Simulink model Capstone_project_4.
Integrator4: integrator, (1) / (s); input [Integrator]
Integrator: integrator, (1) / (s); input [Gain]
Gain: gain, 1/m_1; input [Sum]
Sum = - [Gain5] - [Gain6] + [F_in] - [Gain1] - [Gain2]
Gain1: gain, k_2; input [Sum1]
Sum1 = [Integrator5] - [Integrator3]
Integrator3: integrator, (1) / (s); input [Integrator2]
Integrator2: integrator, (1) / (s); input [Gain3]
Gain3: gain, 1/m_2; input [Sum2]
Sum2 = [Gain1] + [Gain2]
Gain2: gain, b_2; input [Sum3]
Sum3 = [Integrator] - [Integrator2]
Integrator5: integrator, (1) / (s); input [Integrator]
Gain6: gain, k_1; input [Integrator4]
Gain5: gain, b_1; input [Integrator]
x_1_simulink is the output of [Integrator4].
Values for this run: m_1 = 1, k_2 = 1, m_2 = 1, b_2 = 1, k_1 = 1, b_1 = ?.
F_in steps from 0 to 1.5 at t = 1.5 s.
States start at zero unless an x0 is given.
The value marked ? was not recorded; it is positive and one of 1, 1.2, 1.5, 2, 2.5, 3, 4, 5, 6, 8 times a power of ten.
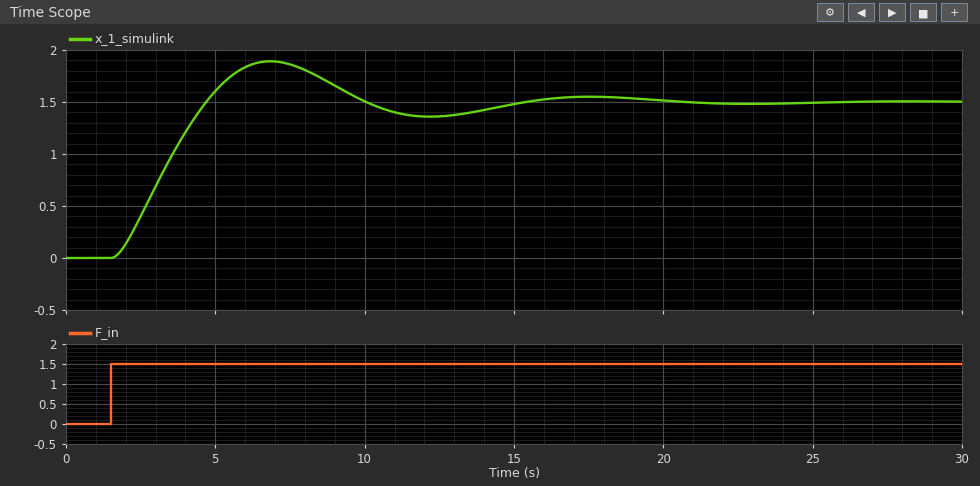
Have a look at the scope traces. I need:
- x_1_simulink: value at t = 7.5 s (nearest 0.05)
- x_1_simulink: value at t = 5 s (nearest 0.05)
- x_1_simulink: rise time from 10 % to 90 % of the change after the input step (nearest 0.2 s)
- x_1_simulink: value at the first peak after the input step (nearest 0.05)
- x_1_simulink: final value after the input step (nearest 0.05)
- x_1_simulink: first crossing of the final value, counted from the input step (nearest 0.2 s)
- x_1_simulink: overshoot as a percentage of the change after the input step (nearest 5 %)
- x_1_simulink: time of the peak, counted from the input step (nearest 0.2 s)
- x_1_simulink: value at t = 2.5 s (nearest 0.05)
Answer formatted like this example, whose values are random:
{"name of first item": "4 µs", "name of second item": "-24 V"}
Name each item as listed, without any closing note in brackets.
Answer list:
{"x_1_simulink: value at t = 7.5 s": "1.85", "x_1_simulink: value at t = 5 s": "1.60", "x_1_simulink: rise time from 10 % to 90 % of the change after the input step": "2.2 s", "x_1_simulink: value at the first peak after the input step": "1.90", "x_1_simulink: final value after the input step": "1.50", "x_1_simulink: first crossing of the final value, counted from the input step": "3.2 s", "x_1_simulink: overshoot as a percentage of the change after the input step": "25 %", "x_1_simulink: time of the peak, counted from the input step": "5.4 s", "x_1_simulink: value at t = 2.5 s": "0.40"}
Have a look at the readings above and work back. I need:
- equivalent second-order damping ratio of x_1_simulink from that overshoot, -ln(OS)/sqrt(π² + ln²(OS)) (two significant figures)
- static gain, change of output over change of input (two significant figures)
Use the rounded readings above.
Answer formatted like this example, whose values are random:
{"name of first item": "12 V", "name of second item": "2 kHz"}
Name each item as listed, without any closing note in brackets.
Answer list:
{"equivalent second-order damping ratio of x_1_simulink from that overshoot, -ln(OS)/sqrt(π² + ln²(OS))": "0.40", "static gain, change of output over change of input": "1.0"}
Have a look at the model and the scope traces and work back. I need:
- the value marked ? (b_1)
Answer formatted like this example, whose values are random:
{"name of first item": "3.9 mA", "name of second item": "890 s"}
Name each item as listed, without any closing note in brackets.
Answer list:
{"the value marked ?": "1"}
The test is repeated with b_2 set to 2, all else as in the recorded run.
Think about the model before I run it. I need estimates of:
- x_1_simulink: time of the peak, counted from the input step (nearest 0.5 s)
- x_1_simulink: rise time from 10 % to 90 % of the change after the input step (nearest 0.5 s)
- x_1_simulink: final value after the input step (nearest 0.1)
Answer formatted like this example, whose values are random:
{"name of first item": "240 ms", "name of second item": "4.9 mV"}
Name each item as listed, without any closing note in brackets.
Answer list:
{"x_1_simulink: time of the peak, counted from the input step": "5.0 s", "x_1_simulink: rise time from 10 % to 90 % of the change after the input step": "2.0 s", "x_1_simulink: final value after the input step": "1.5"}
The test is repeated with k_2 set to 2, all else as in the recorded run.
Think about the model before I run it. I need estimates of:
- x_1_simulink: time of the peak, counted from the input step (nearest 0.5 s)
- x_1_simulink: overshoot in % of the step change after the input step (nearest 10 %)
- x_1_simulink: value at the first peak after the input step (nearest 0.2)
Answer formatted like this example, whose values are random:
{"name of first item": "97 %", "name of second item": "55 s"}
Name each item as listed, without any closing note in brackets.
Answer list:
{"x_1_simulink: time of the peak, counted from the input step": "5.0 s", "x_1_simulink: overshoot in % of the step change after the input step": "30 %", "x_1_simulink: value at the first peak after the input step": "2.0"}
